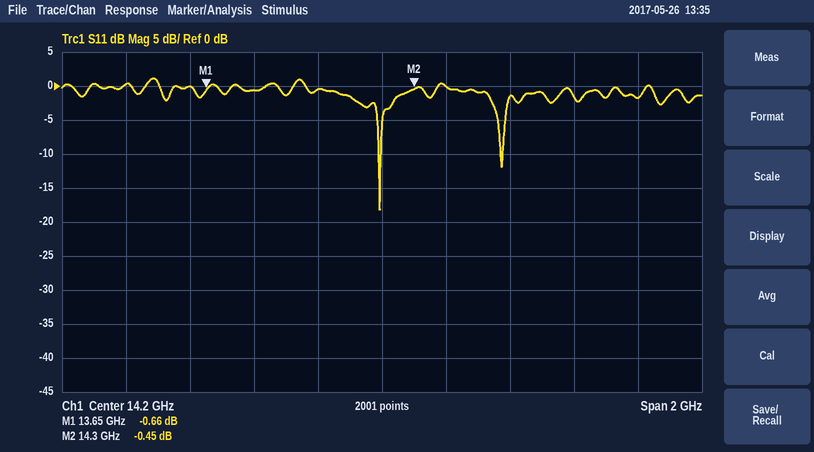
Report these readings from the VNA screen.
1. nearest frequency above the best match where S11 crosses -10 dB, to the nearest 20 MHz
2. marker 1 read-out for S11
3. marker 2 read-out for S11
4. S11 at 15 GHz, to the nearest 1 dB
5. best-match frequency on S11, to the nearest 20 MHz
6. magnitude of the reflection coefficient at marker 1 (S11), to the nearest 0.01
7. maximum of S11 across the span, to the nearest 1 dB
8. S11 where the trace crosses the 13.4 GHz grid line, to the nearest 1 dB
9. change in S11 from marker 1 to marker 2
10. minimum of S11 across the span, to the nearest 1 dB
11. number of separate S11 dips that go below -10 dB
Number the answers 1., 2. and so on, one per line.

1. 14.20 GHz
2. -0.66 dB
3. -0.45 dB
4. -2 dB
5. 14.20 GHz
6. 0.93
7. 1 dB
8. 0 dB
9. 0.21 dB
10. -18 dB
11. 2
